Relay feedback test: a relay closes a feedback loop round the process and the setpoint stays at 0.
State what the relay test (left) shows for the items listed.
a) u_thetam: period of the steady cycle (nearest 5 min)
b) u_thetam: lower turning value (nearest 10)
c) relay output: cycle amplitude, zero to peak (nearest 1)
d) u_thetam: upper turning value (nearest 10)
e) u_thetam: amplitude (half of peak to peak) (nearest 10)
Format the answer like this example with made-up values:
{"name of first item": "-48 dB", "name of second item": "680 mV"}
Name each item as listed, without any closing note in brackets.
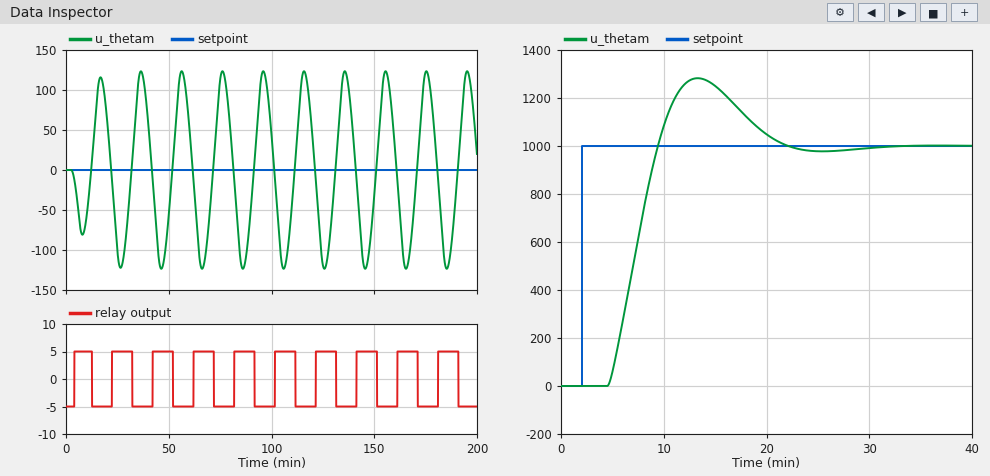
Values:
{"u_thetam: period of the steady cycle": "20 min", "u_thetam: lower turning value": "-120", "relay output: cycle amplitude, zero to peak": "5", "u_thetam: upper turning value": "120", "u_thetam: amplitude (half of peak to peak)": "120"}
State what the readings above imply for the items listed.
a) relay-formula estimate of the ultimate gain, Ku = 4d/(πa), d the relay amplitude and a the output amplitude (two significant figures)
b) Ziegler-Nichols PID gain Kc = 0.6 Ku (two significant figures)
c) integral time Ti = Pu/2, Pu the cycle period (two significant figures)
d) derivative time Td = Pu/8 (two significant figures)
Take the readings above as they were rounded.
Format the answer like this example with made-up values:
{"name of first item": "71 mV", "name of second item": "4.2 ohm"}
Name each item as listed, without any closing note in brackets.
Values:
{"relay-formula estimate of the ultimate gain, Ku = 4d/(πa), d the relay amplitude and a the output amplitude": "0.053", "Ziegler-Nichols PID gain Kc = 0.6 Ku": "0.032", "integral time Ti = Pu/2, Pu the cycle period": "10 min", "derivative time Td = Pu/8": "2.5 min"}
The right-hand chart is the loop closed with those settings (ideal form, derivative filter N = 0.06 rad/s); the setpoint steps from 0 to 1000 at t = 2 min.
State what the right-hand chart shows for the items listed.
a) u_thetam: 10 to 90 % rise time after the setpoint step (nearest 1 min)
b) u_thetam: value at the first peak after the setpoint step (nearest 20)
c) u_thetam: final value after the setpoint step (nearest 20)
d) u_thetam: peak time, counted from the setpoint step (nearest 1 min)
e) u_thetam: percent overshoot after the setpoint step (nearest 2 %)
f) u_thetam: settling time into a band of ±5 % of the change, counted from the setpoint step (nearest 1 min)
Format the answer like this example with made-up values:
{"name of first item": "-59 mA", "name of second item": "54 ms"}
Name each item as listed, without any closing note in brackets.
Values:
{"u_thetam: 10 to 90 % rise time after the setpoint step": "4 min", "u_thetam: value at the first peak after the setpoint step": "1280", "u_thetam: final value after the setpoint step": "1000", "u_thetam: peak time, counted from the setpoint step": "11 min", "u_thetam: percent overshoot after the setpoint step": "28 %", "u_thetam: settling time into a band of ±5 % of the change, counted from the setpoint step": "18 min"}
